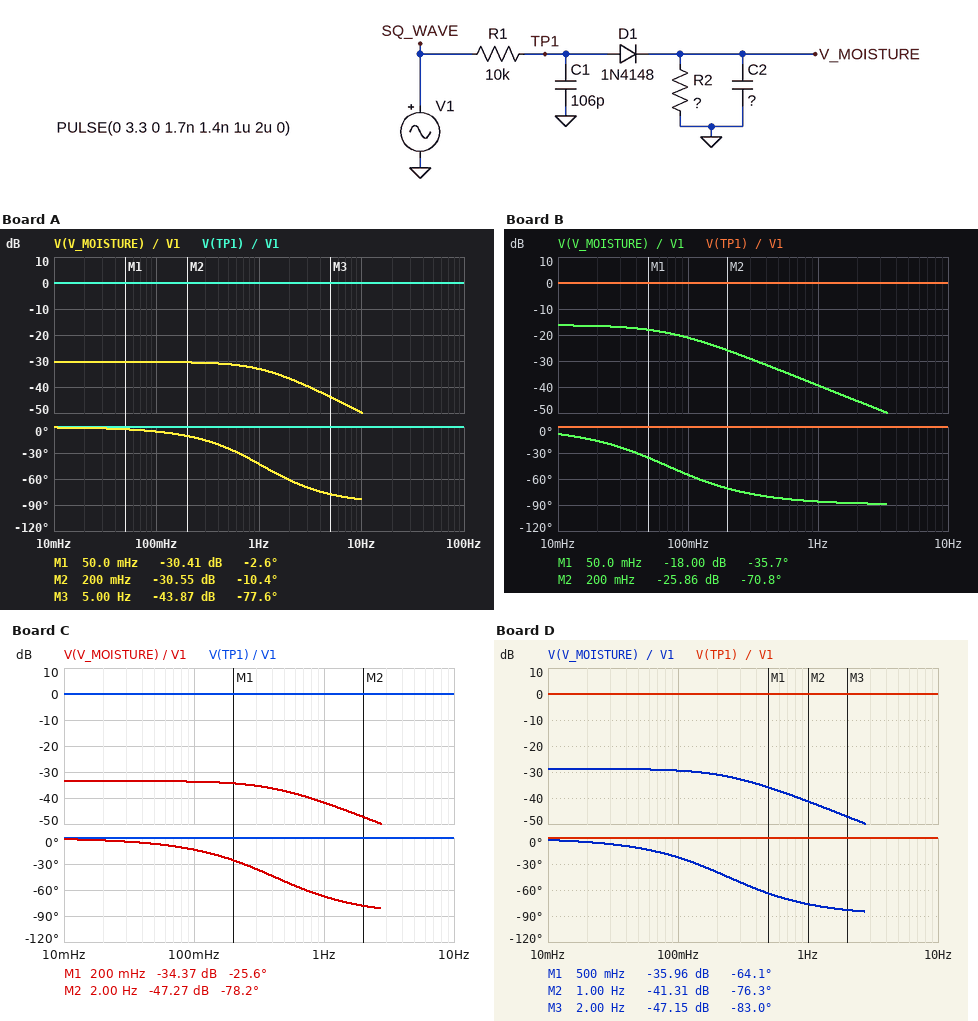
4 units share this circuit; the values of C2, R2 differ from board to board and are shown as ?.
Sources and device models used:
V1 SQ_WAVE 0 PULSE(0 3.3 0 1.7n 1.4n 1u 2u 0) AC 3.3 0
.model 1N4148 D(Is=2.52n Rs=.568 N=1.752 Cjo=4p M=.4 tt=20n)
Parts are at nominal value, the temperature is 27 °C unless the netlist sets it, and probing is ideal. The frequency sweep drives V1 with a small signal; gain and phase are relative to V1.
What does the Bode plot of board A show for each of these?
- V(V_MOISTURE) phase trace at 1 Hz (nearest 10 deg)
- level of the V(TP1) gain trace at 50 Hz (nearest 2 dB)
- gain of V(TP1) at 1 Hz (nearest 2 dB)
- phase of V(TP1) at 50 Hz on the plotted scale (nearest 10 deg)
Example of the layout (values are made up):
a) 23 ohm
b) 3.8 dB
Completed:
a) -40 deg
b) 0 dB
c) 0 dB
d) 0 deg
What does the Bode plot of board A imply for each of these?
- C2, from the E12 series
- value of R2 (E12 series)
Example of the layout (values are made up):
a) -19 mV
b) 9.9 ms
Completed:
a) 270 nF
b) 560 kΩ
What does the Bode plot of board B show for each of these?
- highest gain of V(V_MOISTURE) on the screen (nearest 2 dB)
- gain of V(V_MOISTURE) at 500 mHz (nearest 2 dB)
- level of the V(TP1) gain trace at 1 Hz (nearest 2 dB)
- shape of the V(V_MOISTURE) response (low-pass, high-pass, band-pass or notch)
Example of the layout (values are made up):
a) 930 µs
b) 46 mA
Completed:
a) -16 dB
b) -34 dB
c) 0 dB
d) low-pass
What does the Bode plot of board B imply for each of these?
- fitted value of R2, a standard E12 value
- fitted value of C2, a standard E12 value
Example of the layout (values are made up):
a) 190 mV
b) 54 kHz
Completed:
a) 3.3 MΩ
b) 820 nF
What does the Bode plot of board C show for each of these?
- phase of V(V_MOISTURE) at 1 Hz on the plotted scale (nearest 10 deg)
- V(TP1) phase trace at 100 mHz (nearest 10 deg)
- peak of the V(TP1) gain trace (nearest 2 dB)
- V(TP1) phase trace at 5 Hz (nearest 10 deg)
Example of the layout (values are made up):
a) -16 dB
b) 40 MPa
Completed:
a) -70 deg
b) 0 deg
c) 0 dB
d) 0 deg
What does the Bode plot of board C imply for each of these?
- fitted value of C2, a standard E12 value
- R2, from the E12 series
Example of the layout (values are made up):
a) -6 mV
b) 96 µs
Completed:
a) 1 µF
b) 390 kΩ
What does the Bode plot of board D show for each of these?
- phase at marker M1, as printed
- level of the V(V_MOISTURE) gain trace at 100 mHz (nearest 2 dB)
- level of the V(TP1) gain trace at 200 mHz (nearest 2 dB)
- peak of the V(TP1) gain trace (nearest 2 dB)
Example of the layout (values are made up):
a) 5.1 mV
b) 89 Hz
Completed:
a) -64.1 deg
b) -30 dB
c) 0 dB
d) 0 dB
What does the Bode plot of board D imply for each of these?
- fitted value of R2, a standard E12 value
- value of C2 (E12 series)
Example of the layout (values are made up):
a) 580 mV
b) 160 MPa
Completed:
a) 680 kΩ
b) 1 µF
